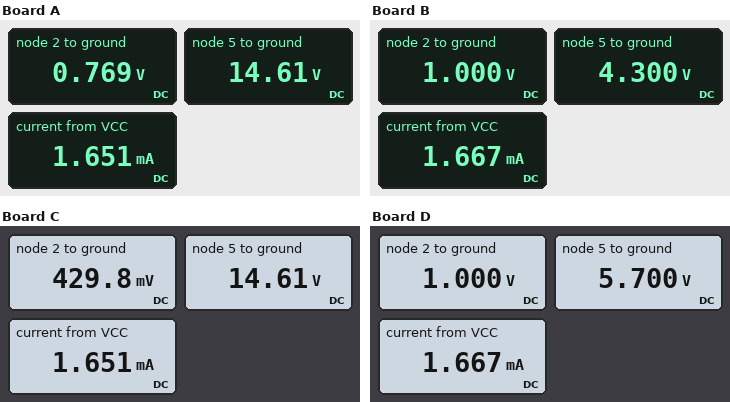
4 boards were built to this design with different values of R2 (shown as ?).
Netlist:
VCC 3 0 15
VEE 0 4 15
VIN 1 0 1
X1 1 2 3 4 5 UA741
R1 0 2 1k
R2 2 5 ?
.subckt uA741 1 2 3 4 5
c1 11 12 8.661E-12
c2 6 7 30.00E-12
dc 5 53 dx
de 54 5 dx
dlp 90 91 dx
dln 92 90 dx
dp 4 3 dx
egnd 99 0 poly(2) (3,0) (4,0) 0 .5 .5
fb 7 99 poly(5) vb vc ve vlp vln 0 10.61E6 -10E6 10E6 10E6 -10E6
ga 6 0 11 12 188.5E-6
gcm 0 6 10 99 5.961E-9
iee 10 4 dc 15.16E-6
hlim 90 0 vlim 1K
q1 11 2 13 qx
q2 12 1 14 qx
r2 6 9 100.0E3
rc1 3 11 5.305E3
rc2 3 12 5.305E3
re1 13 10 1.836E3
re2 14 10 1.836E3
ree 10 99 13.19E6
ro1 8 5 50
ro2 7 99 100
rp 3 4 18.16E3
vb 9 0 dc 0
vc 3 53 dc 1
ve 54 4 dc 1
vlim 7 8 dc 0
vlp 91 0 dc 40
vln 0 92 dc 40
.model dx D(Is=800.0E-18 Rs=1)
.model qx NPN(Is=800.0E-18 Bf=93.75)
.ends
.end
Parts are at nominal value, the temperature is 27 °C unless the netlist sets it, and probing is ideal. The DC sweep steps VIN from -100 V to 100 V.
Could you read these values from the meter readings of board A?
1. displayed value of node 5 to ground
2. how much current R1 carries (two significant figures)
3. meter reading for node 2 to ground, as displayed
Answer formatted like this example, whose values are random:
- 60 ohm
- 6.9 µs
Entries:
- 14.61 V
- 770 µA
- 0.769 V
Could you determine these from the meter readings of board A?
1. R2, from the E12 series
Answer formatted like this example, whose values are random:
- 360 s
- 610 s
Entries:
- 18 kΩ
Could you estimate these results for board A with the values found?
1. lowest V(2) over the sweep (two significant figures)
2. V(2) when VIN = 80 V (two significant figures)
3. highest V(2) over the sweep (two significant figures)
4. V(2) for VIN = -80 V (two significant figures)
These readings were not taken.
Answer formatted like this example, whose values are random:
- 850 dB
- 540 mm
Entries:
- -780 mV
- -780 mV
- 770 mV
- -770 mV
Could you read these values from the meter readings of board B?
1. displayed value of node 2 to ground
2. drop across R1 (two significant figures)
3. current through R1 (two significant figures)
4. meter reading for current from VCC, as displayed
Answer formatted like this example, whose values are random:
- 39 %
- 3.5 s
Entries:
- 1.000 V
- 1.0 V
- 1.0 mA
- 1.667 mA
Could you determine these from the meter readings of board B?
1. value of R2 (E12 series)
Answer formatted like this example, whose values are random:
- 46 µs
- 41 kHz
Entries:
- 3.3 kΩ
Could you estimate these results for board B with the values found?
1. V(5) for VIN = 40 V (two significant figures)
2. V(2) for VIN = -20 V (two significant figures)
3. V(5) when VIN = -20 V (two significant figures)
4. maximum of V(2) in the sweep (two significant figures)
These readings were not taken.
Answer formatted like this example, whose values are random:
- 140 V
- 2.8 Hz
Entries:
- -15 V
- -3.4 V
- -15 V
- 3.4 V
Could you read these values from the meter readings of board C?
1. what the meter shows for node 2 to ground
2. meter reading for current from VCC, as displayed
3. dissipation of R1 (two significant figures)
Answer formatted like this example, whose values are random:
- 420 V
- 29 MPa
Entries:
- 429.8 mV
- 1.651 mA
- 180 µW
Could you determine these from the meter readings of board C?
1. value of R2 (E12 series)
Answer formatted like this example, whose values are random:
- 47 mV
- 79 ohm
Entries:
- 33 kΩ
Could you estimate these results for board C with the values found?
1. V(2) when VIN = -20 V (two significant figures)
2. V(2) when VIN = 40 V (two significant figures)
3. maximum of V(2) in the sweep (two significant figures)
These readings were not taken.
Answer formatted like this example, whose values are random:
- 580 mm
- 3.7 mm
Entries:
- -430 mV
- -430 mV
- 430 mV
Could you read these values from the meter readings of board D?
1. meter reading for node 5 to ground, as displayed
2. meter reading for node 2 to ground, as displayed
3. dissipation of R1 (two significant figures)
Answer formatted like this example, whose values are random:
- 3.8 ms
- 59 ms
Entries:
- 5.700 V
- 1.000 V
- 1.0 mW
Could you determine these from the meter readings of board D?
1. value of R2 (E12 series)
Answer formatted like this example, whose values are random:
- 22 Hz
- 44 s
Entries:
- 4.7 kΩ
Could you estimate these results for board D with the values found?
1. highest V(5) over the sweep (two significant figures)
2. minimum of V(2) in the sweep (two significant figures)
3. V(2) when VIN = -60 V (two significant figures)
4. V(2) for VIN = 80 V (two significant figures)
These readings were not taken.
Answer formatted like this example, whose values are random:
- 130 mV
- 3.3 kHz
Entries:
- 15 V
- -2.6 V
- -2.6 V
- -2.6 V
